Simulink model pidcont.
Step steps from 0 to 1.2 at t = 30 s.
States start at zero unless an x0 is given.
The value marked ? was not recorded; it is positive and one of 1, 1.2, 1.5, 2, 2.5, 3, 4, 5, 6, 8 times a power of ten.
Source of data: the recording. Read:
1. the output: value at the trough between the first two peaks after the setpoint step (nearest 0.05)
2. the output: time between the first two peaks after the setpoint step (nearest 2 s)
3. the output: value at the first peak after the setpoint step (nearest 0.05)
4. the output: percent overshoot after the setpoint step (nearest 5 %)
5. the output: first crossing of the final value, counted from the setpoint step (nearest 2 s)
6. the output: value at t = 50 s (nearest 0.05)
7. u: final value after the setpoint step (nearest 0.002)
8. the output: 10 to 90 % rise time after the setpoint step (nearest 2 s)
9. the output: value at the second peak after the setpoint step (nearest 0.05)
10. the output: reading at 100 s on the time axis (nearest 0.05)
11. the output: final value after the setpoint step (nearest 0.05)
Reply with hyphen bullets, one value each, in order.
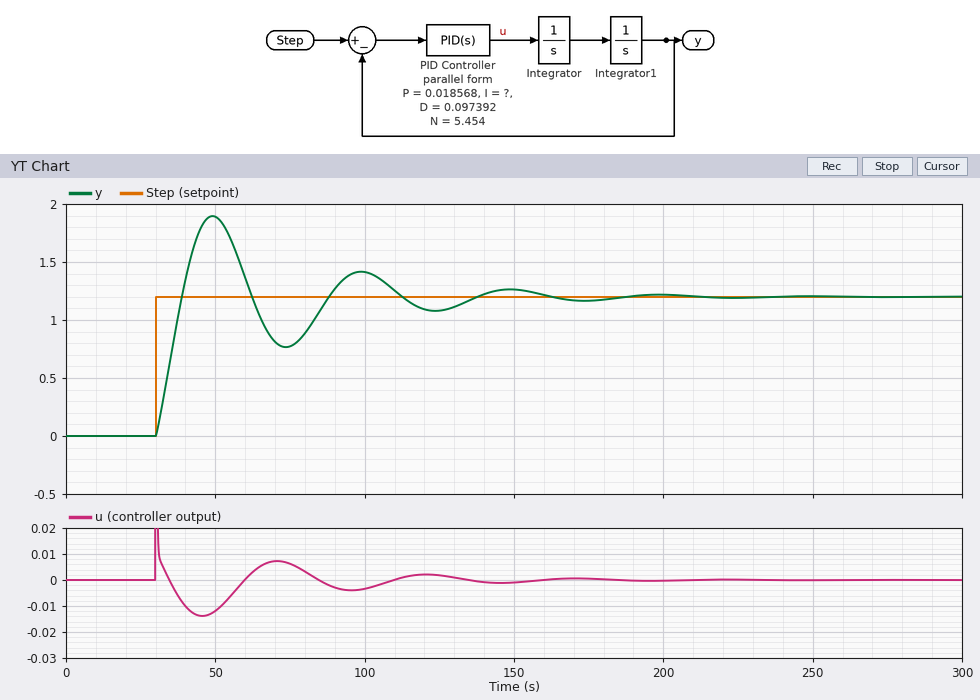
- 0.75
- 50 s
- 1.90
- 60 %
- 8 s
- 1.90
- 0.000
- 6 s
- 1.40
- 1.40
- 1.20
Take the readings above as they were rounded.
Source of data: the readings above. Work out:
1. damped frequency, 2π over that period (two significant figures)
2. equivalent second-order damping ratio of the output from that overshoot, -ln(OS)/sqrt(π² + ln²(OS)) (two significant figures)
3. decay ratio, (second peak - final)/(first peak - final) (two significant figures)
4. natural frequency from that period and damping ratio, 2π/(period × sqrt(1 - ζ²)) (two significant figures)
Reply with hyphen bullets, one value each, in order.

- 0.13 rad/s
- 0.16
- 0.29
- 0.13 rad/s
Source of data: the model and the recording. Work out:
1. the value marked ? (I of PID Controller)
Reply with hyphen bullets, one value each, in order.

- 0.0008
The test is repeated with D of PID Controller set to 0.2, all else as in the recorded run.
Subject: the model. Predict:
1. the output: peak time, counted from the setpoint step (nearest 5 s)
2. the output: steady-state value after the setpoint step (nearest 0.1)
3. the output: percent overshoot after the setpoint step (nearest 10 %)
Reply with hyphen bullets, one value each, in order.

- 15 s
- 1.2
- 30 %
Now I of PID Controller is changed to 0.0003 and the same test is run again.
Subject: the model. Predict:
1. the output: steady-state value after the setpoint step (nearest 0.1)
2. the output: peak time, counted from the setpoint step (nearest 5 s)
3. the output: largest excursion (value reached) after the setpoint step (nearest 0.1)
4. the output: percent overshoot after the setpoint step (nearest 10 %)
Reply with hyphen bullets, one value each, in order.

- 1.2
- 20 s
- 1.8
- 50 %
